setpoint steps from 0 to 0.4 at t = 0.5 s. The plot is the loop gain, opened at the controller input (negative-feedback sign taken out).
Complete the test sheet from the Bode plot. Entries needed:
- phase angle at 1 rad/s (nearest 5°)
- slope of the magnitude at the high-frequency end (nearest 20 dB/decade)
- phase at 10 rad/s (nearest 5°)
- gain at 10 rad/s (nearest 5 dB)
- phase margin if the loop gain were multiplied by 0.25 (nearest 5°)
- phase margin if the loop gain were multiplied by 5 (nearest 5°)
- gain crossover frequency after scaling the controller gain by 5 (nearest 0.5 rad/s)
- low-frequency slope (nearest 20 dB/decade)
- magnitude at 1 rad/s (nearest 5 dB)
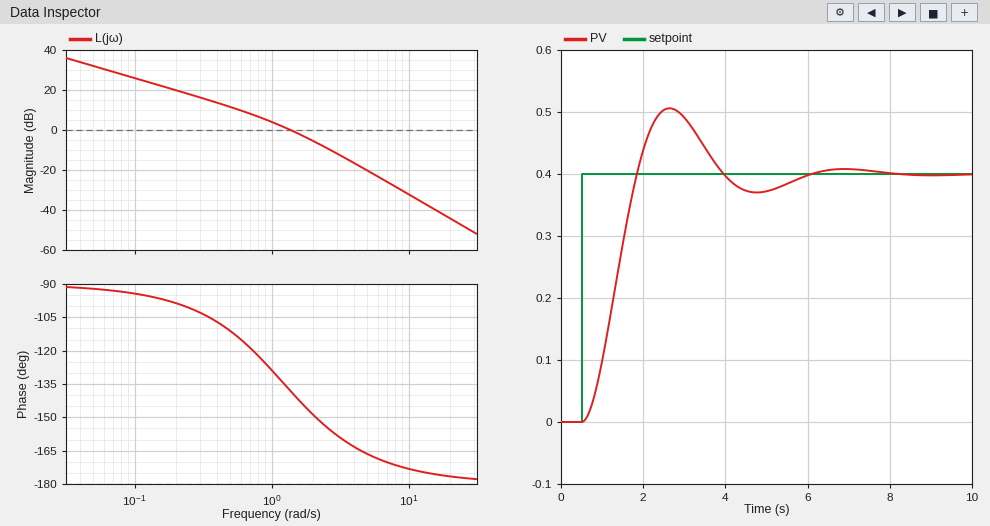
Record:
-130°
-40 dB/decade
-175°
-30 dB
70°
20°
3.5 rad/s
-20 dB/decade
5 dB
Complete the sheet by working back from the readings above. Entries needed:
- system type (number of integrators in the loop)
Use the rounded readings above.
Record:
1
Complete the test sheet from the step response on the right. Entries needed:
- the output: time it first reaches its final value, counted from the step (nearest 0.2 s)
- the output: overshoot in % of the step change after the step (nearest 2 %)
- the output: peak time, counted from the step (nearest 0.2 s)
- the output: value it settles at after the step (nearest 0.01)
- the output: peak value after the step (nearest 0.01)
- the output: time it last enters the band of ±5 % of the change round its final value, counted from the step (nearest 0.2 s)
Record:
1.4 s
26 %
2.2 s
0.40
0.51
4.8 s
